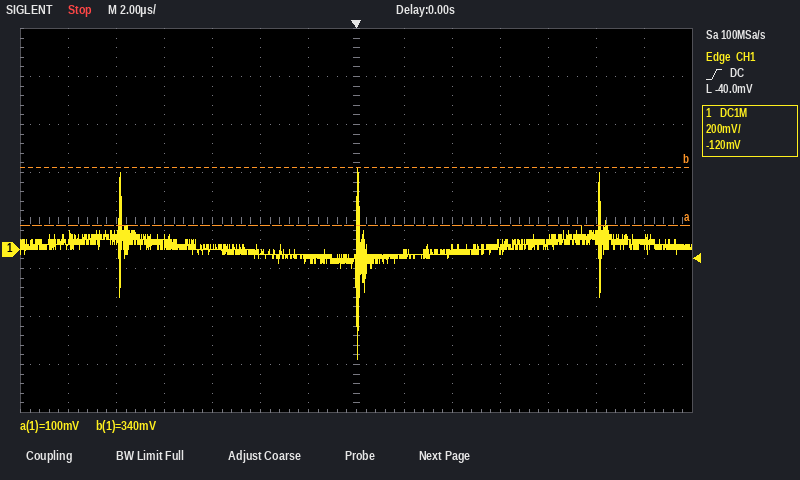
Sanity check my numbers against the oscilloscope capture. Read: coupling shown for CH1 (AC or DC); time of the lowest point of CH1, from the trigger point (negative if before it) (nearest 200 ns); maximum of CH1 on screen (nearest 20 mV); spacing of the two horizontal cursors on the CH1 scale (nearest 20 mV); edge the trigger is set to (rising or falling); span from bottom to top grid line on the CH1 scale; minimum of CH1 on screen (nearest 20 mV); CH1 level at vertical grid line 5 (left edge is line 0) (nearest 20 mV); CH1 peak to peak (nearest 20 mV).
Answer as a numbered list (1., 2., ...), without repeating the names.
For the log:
1. DC
2. 0.0 µs
3. 340 mV
4. 240 mV
5. rising
6. 1.6 V
7. -460 mV
8. -20 mV
9. 800 mV
